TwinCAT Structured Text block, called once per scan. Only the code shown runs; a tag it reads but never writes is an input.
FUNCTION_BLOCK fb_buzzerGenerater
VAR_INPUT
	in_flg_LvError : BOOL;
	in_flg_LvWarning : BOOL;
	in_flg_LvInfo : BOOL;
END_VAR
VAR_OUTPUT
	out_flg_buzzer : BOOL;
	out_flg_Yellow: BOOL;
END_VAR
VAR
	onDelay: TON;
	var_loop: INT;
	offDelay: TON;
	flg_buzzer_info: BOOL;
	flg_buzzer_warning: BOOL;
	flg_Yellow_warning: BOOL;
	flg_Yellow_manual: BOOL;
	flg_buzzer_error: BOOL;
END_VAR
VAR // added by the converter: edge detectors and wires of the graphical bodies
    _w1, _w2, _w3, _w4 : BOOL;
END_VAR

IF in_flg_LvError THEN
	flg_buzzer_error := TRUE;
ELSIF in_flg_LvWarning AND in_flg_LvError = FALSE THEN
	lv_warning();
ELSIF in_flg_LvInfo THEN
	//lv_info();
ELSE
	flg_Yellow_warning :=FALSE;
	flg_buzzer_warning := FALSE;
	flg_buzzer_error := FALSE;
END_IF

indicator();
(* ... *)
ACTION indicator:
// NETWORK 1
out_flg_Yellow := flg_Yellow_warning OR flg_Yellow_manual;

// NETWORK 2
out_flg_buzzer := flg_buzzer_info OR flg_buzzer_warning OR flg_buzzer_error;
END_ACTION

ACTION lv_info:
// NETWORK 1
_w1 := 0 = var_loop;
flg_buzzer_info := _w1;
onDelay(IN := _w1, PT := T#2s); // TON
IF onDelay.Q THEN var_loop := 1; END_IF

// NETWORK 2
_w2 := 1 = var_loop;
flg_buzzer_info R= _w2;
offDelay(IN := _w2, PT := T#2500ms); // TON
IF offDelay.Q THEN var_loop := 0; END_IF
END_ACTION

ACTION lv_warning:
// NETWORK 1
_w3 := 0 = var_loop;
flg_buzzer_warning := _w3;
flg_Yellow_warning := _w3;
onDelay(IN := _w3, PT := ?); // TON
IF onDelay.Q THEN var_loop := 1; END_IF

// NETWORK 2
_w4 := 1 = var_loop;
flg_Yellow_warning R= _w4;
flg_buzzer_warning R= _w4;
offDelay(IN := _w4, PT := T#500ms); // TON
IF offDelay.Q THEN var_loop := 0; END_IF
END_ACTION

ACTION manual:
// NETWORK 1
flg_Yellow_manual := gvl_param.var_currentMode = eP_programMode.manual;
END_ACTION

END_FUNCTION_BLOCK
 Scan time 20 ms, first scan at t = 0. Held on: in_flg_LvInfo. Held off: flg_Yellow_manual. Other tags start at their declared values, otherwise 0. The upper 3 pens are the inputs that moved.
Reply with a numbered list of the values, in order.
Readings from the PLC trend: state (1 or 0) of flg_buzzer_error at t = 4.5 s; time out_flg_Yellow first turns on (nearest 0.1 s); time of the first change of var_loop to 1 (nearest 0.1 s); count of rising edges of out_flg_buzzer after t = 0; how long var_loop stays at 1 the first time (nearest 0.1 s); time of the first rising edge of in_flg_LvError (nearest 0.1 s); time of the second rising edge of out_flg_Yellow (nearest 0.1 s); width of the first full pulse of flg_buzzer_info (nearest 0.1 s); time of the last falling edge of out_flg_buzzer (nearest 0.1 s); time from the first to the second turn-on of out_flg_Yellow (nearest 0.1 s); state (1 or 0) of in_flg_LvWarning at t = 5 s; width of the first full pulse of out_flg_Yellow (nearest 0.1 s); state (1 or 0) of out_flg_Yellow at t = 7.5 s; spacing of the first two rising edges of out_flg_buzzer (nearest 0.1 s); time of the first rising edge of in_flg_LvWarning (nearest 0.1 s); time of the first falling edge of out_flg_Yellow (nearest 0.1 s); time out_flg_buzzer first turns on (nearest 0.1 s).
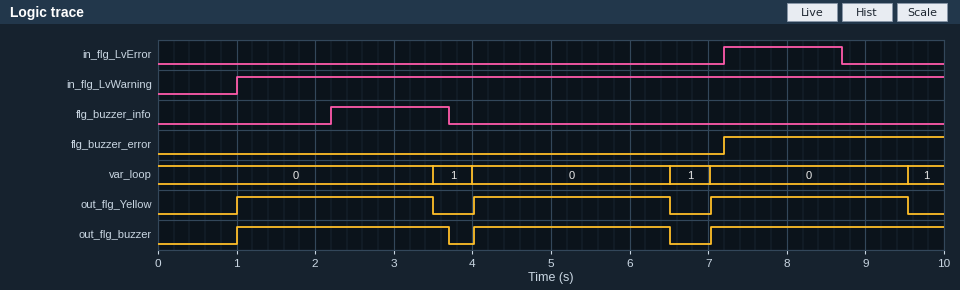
1. 0
2. 1.0 s
3. 3.5 s
4. 3
5. 0.5 s
6. 7.2 s
7. 4.0 s
8. 1.5 s
9. 6.5 s
10. 3.0 s
11. 1
12. 2.5 s
13. 1
14. 3.0 s
15. 1.0 s
16. 3.5 s
17. 1.0 s
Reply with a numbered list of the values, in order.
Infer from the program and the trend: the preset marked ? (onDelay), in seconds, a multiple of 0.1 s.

1. 2.5 s
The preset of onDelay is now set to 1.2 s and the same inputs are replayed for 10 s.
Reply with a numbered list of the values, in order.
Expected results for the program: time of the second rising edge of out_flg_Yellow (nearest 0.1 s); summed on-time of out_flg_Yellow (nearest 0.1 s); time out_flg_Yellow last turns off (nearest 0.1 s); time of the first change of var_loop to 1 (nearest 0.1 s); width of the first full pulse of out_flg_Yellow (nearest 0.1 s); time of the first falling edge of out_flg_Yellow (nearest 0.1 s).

1. 2.7 s
2. 6.9 s
3. 8.7 s
4. 2.2 s
5. 1.2 s
6. 2.2 s
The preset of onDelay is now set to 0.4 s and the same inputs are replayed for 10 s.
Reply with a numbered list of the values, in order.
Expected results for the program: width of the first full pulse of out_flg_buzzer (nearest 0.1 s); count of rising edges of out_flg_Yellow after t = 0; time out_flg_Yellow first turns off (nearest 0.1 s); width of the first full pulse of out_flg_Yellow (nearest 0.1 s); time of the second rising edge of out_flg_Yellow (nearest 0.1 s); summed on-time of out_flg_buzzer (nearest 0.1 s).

1. 0.4 s
2. 9
3. 1.4 s
4. 0.4 s
5. 1.9 s
6. 6.6 s
